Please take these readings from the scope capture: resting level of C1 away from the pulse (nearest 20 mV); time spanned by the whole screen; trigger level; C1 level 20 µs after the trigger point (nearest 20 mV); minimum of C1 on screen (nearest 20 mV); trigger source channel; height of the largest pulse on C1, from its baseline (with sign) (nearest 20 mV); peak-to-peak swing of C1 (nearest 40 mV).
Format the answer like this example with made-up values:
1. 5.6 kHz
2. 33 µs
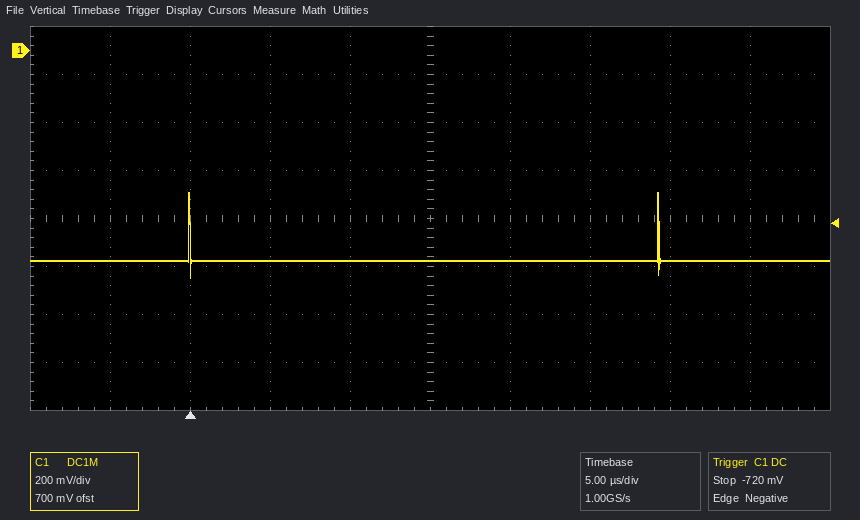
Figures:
1. -880 mV
2. 50 µs
3. -720 mV
4. -880 mV
5. -940 mV
6. C1
7. +280 mV
8. 360 mV
